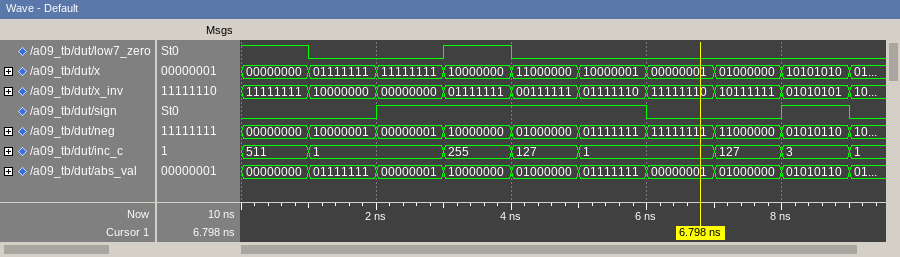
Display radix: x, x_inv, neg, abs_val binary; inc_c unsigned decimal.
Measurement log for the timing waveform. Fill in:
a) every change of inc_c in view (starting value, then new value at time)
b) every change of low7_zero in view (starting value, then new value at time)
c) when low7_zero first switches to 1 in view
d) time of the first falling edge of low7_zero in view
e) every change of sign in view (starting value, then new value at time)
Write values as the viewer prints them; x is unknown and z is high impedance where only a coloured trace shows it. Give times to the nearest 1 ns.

511, 1 at 1 ns, 255 at 3 ns, 127 at 4 ns, 1 at 5 ns, 127 at 7 ns, 3 at 8 ns, 1 at 9 ns
1, 0 at 1 ns, 1 at 3 ns, 0 at 4 ns
3 ns
1 ns
0, 1 at 2 ns, 0 at 6 ns, 1 at 8 ns, 0 at 9 ns
